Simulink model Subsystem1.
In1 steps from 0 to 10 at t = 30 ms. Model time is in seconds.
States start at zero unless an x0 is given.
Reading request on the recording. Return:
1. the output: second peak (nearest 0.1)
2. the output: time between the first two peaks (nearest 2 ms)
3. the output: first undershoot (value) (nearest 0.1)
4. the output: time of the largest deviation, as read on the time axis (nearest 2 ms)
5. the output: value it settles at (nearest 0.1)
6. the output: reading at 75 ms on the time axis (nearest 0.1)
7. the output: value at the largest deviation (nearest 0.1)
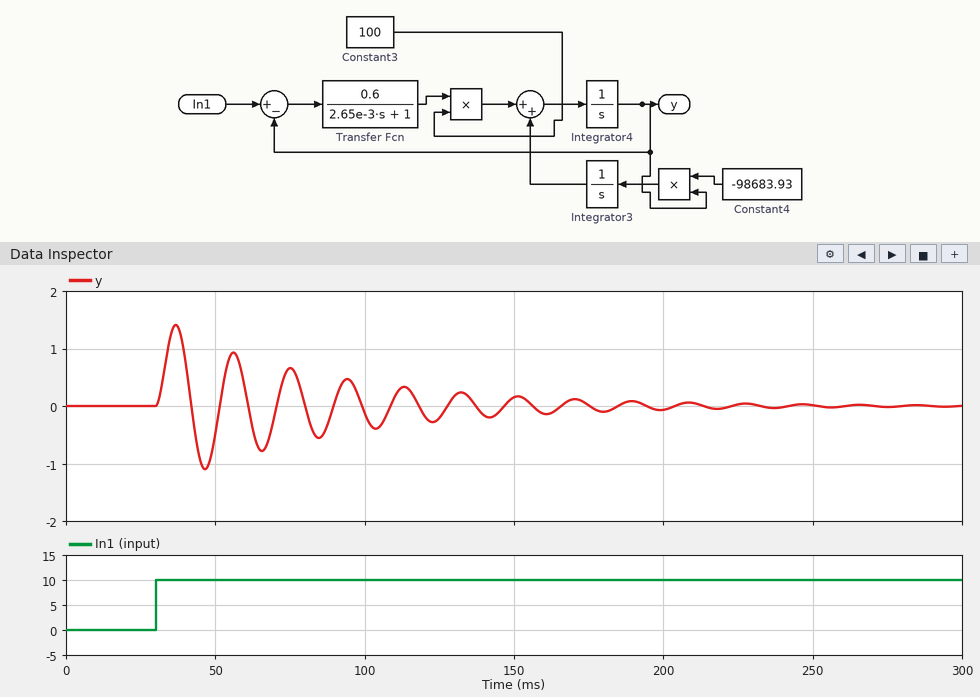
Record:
0.9
20 ms
-1.1
36 ms
0.0
0.7
1.4
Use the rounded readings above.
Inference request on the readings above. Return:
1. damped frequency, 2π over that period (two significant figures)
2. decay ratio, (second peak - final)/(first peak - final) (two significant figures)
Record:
0.31 rad/ms
0.64
